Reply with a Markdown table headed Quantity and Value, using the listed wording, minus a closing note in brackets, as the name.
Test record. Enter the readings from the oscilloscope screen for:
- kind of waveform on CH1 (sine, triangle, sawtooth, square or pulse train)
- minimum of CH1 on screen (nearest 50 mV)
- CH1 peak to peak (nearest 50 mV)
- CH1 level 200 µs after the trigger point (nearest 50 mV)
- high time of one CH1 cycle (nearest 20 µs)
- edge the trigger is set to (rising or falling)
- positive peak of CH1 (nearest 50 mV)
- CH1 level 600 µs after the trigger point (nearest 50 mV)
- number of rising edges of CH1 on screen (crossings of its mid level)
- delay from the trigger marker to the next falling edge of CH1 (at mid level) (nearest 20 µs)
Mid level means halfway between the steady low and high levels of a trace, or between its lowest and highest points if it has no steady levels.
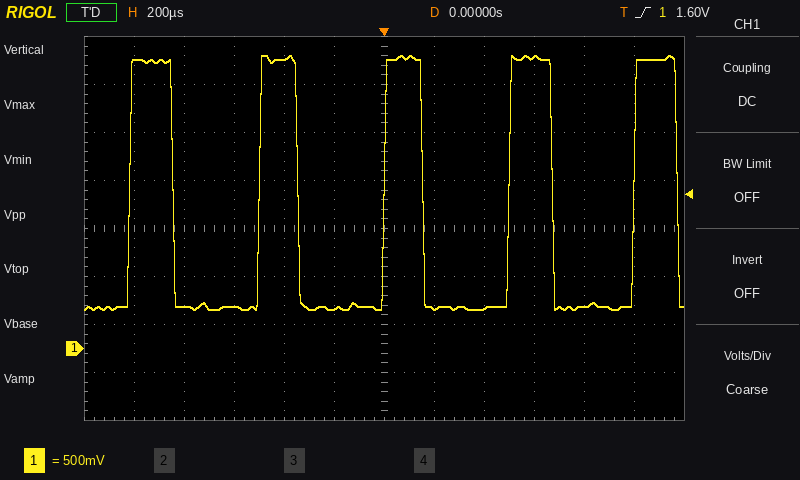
| Quantity | Value |
|---|---|
| kind of waveform on CH1 | pulse train |
| minimum of CH1 on screen | 400 mV |
| CH1 peak to peak | 2.65 V |
| CH1 level 200 µs after the trigger point | 400 mV |
| high time of one CH1 cycle | 160 µs |
| edge the trigger is set to | rising |
| positive peak of CH1 | 3.05 V |
| CH1 level 600 µs after the trigger point | 3.05 V |
| number of rising edges of CH1 on screen | 5 |
| delay from the trigger marker to the next falling edge of CH1 (at mid level) | 160 µs |
